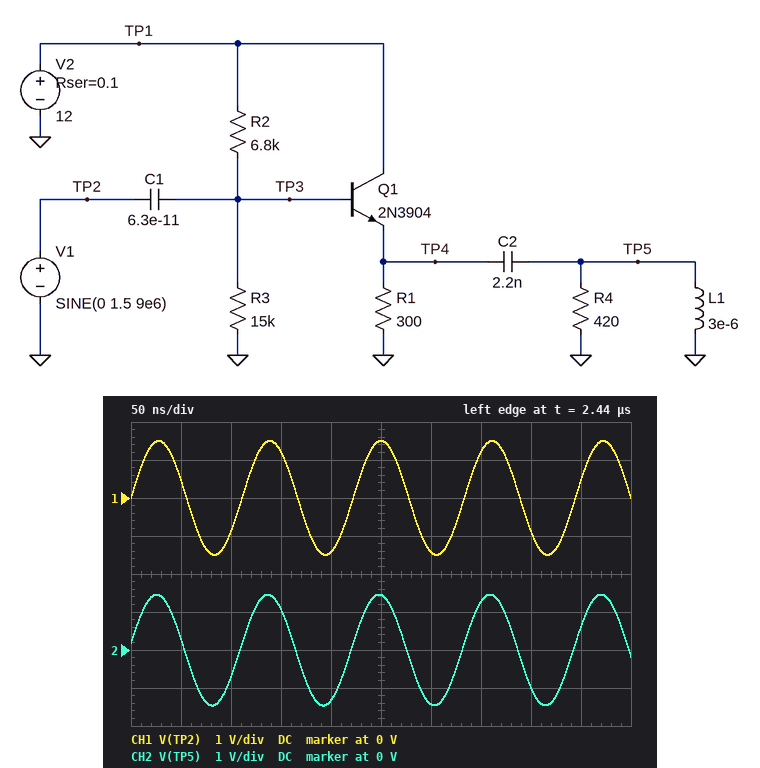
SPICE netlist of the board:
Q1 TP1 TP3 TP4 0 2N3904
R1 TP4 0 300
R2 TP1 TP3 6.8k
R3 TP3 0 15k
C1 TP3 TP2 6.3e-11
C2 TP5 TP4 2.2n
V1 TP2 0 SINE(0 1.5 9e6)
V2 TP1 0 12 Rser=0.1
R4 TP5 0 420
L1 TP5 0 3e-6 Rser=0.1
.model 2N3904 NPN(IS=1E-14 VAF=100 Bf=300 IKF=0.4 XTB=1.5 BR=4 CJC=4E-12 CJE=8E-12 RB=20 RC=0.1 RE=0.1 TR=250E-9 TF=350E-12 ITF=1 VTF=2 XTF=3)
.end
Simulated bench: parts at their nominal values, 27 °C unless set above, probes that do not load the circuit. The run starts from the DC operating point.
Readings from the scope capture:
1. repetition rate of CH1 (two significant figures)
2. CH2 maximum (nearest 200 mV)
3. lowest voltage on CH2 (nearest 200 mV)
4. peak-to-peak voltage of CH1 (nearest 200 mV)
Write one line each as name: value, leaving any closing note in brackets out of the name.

repetition rate of CH1: 9.0 MHz
CH2 maximum: 1.4 V
lowest voltage on CH2: -1.4 V
peak-to-peak voltage of CH1: 3.0 V
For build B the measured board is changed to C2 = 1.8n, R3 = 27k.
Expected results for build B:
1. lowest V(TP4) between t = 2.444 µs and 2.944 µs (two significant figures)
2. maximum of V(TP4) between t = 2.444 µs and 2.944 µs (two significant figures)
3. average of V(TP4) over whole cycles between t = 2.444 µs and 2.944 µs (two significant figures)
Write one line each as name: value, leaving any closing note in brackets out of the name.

lowest V(TP4) between t = 2.444 µs and 2.944 µs: 6.9 V
maximum of V(TP4) between t = 2.444 µs and 2.944 µs: 9.7 V
average of V(TP4) over whole cycles between t = 2.444 µs and 2.944 µs: 8.3 V
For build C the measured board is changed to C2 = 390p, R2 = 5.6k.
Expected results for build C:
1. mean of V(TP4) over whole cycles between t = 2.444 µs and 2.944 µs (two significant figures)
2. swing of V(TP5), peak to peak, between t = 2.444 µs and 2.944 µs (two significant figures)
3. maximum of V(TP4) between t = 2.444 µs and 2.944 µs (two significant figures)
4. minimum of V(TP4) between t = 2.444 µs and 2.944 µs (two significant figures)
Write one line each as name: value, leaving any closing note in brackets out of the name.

mean of V(TP4) over whole cycles between t = 2.444 µs and 2.944 µs: 7.6 V
swing of V(TP5), peak to peak, between t = 2.444 µs and 2.944 µs: 3.7 V
maximum of V(TP4) between t = 2.444 µs and 2.944 µs: 9.0 V
minimum of V(TP4) between t = 2.444 µs and 2.944 µs: 6.3 V
